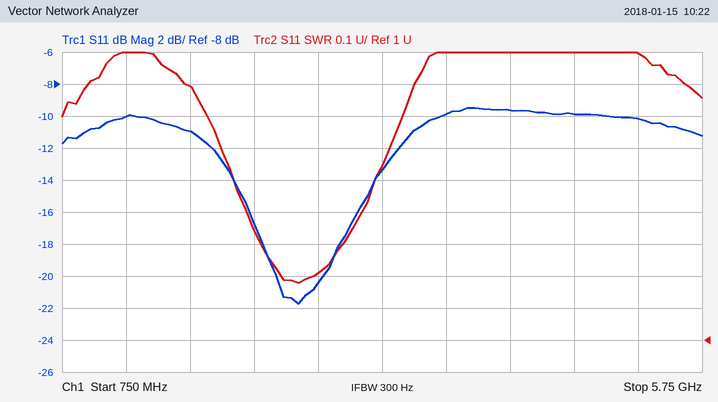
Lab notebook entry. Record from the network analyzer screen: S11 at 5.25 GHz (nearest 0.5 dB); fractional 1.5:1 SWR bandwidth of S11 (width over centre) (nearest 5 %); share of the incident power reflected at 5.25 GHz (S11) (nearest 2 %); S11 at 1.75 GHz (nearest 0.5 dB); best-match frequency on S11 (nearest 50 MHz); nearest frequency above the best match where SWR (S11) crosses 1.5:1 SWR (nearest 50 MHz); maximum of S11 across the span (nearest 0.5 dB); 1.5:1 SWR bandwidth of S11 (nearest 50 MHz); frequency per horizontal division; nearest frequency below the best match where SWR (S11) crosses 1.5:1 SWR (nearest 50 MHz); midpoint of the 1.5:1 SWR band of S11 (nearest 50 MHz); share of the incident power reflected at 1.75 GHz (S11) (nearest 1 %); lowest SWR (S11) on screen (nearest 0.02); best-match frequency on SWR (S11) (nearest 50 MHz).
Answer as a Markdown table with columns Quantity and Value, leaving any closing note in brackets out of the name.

| Quantity | Value |
|---|---|
| S11 at 5.25 GHz | -10.0 dB |
| fractional 1.5:1 SWR bandwidth of S11 (width over centre) | 40 % |
| share of the incident power reflected at 5.25 GHz (S11) | 10 % |
| S11 at 1.75 GHz | -11.0 dB |
| best-match frequency on S11 | 2.60 GHz |
| nearest frequency above the best match where SWR (S11) crosses 1.5:1 SWR | 3.20 GHz |
| maximum of S11 across the span | -9.5 dB |
| 1.5:1 SWR bandwidth of S11 | 1.10 GHz |
| frequency per horizontal division | 500 MHz |
| nearest frequency below the best match where SWR (S11) crosses 1.5:1 SWR | 2.10 GHz |
| midpoint of the 1.5:1 SWR band of S11 | 2.65 GHz |
| share of the incident power reflected at 1.75 GHz (S11) | 8 % |
| lowest SWR (S11) on screen | 1.18 |
| best-match frequency on SWR (S11) | 2.60 GHz |
